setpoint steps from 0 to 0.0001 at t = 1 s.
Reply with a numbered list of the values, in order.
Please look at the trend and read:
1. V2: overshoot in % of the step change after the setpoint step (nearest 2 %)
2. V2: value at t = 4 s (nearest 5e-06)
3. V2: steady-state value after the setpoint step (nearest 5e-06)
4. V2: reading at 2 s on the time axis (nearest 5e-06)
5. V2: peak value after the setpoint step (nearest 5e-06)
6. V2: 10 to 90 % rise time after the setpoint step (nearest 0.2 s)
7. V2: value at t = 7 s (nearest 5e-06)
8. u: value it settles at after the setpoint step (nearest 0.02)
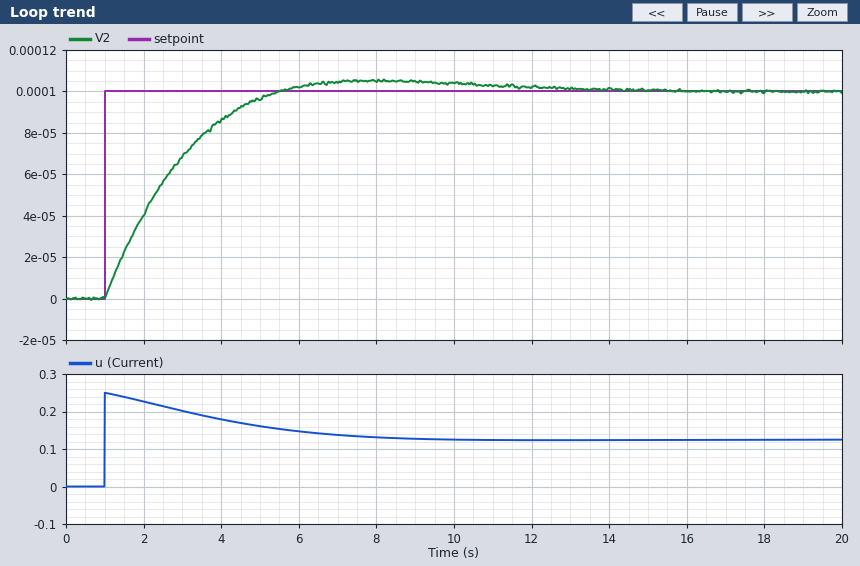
1. 6 %
2. 0.000085
3. 0.000100
4. 0.000040
5. 0.000105
6. 3.0 s
7. 0.000105
8. 0.12
